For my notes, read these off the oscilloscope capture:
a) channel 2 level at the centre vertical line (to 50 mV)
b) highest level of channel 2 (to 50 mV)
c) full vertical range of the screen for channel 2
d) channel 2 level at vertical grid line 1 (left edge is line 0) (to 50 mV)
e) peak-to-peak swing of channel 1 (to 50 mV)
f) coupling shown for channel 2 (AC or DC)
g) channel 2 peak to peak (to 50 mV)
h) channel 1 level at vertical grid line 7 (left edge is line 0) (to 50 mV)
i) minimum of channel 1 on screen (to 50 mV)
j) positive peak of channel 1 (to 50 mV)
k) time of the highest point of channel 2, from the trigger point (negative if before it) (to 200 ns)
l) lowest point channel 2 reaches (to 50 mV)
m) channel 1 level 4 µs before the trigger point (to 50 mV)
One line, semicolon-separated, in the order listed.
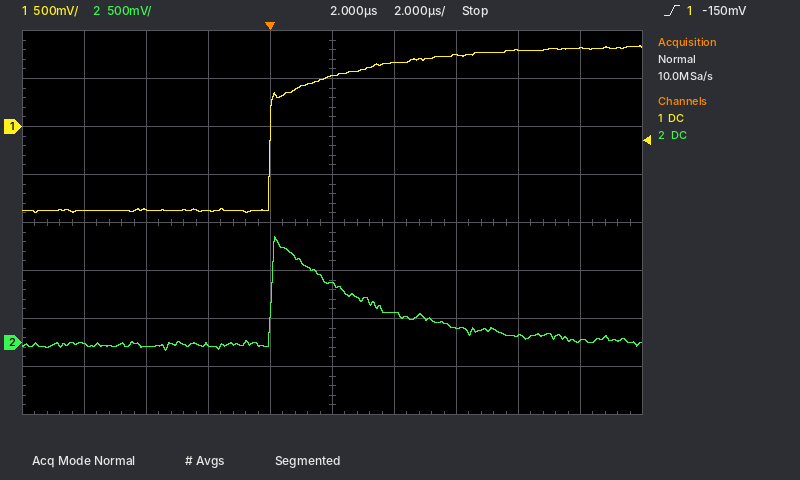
600 mV; 1.10 V; 4 V; 0 mV; 1.75 V; DC; 1.20 V; 750 mV; -900 mV; 850 mV; +200 ns; -100 mV; -850 mV
